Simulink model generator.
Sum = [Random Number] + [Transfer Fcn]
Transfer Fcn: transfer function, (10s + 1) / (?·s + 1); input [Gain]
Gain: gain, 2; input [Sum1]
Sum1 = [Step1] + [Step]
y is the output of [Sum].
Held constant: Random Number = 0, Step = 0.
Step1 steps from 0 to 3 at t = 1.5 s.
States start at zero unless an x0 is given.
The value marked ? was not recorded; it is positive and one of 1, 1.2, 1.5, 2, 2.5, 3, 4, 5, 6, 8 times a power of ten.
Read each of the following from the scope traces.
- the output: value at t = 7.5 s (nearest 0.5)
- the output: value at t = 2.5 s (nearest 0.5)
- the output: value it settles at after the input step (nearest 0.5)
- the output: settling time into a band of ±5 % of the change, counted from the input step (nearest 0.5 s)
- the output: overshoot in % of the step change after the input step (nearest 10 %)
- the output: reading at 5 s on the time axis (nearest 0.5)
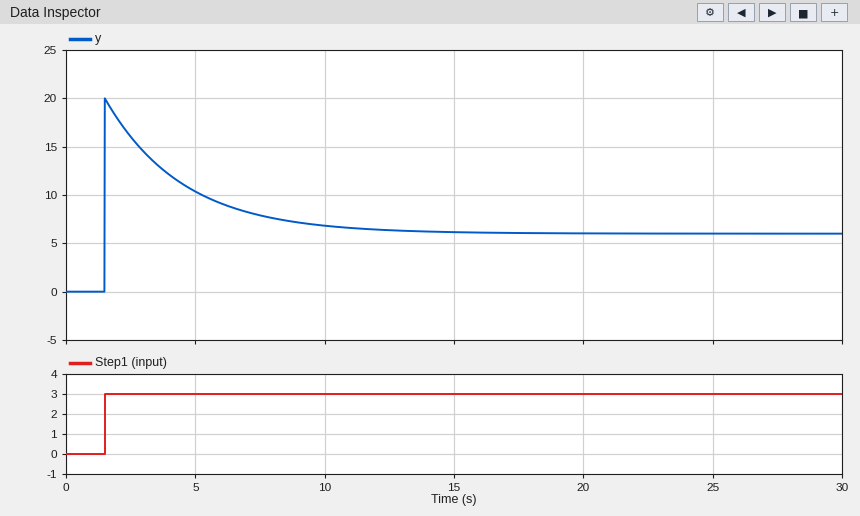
8.0
16.0
6.0
11.5 s
230 %
10.5
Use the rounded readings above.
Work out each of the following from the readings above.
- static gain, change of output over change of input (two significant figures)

2.0
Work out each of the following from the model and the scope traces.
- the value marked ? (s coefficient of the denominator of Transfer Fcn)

3
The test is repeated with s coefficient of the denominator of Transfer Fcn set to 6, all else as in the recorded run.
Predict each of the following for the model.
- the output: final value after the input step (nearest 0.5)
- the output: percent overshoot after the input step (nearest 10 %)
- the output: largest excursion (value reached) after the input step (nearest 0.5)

6.0
70 %
10.0
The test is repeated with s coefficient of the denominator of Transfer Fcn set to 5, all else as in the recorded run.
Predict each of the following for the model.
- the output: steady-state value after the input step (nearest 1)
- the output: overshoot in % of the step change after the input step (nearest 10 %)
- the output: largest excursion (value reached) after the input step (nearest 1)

6
100 %
12
